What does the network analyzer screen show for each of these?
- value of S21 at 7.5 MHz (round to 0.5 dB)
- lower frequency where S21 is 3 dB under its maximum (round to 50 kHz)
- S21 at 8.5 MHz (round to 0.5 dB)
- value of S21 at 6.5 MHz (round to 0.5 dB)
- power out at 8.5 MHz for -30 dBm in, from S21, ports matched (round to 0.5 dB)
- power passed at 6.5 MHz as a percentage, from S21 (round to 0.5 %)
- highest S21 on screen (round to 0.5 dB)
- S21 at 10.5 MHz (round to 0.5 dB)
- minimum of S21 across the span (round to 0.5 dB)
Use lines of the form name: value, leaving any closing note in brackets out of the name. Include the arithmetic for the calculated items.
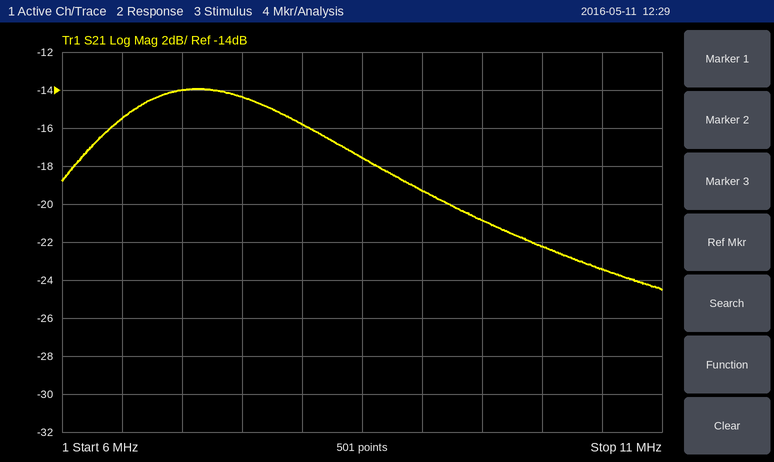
value of S21 at 7.5 MHz: -14.5 dB
lower frequency where S21 is 3 dB under its maximum: 6.25 MHz
S21 at 8.5 MHz: -17.5 dB
value of S21 at 6.5 MHz: -15.5 dB
power out at 8.5 MHz for -30 dBm in, from S21, ports matched: -30 dBm + (-17.5 dB) = -47.5 dBm
power passed at 6.5 MHz as a percentage, from S21: 10^(-15.5/10) ≈ 2.82 %, so 3.0 % to the nearest 0.5 %
highest S21 on screen: -14.0 dB
S21 at 10.5 MHz: -23.5 dB
minimum of S21 across the span: -24.5 dB
